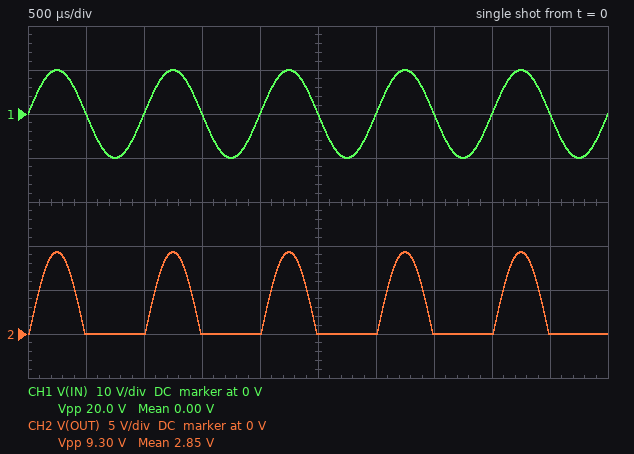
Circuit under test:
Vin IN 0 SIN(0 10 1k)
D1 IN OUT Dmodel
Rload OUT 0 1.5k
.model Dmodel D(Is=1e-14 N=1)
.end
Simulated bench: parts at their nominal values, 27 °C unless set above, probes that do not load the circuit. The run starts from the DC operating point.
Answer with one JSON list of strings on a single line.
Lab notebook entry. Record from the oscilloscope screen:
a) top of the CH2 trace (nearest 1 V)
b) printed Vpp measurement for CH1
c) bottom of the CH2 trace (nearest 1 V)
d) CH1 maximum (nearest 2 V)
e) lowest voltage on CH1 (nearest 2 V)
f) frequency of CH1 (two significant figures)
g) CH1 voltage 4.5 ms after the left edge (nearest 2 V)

["9 V", "20.0 V", "0 V", "10 V", "-10 V", "1.0 kHz", "0 V"]
